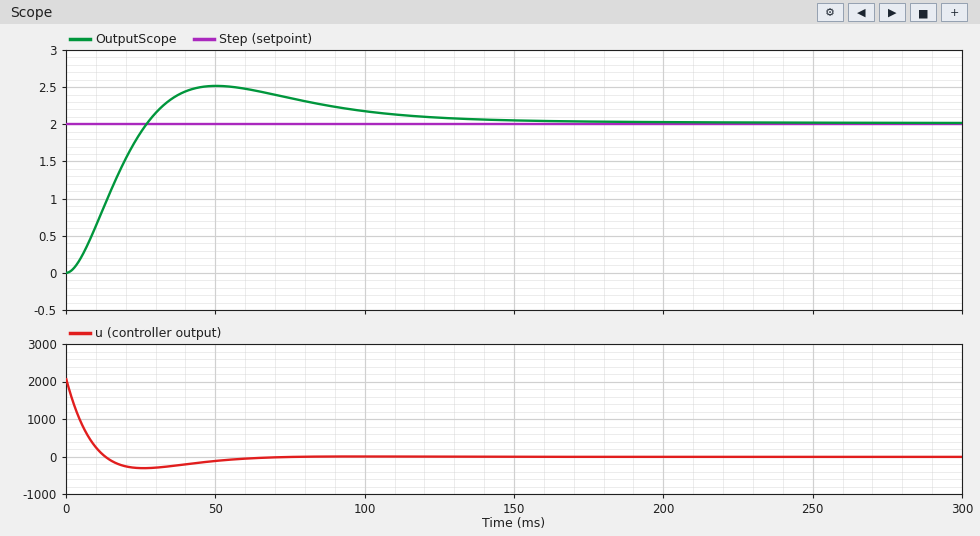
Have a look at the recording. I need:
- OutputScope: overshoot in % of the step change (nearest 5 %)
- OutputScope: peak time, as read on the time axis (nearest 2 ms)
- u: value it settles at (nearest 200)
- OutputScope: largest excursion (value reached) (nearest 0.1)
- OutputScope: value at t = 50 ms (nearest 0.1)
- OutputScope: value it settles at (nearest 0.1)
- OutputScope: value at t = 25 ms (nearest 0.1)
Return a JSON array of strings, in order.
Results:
["25 %", "50 ms", "0", "2.5", "2.5", "2.0", "1.9"]
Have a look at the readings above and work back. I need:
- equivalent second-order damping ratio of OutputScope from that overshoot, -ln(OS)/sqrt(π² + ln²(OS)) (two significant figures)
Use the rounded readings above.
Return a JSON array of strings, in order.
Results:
["0.40"]
